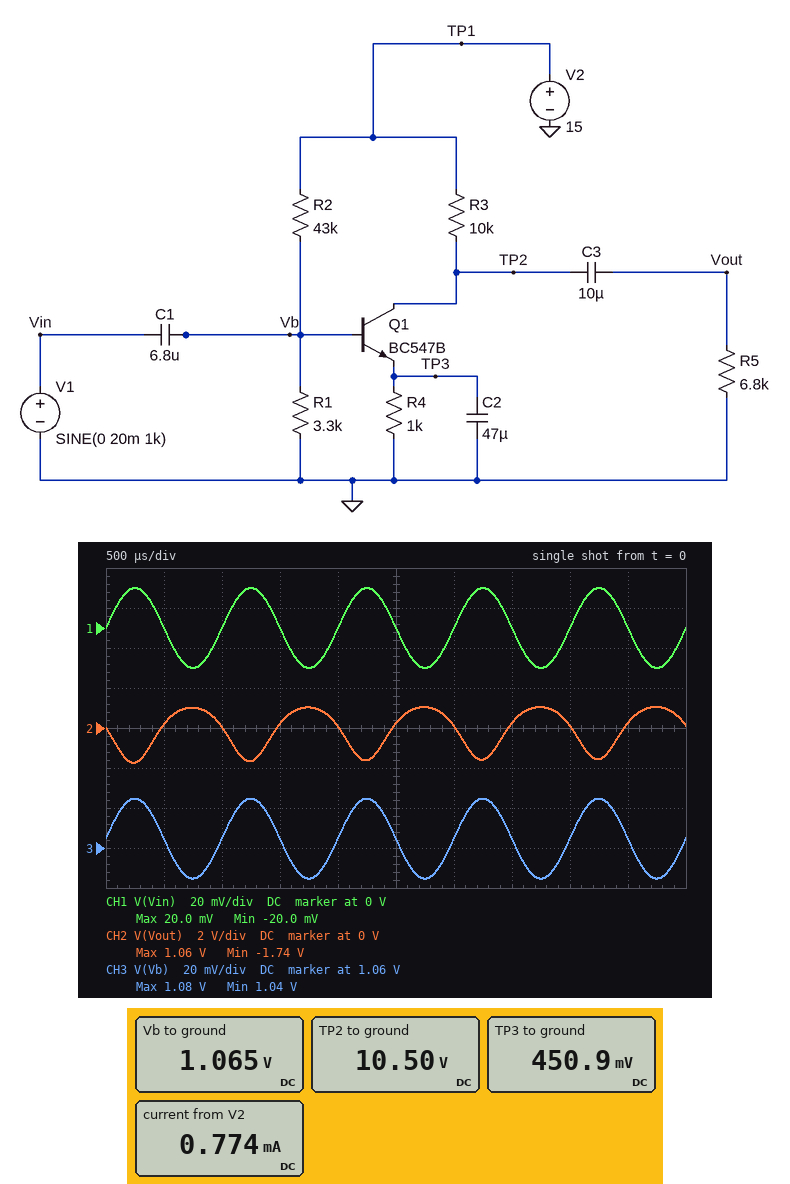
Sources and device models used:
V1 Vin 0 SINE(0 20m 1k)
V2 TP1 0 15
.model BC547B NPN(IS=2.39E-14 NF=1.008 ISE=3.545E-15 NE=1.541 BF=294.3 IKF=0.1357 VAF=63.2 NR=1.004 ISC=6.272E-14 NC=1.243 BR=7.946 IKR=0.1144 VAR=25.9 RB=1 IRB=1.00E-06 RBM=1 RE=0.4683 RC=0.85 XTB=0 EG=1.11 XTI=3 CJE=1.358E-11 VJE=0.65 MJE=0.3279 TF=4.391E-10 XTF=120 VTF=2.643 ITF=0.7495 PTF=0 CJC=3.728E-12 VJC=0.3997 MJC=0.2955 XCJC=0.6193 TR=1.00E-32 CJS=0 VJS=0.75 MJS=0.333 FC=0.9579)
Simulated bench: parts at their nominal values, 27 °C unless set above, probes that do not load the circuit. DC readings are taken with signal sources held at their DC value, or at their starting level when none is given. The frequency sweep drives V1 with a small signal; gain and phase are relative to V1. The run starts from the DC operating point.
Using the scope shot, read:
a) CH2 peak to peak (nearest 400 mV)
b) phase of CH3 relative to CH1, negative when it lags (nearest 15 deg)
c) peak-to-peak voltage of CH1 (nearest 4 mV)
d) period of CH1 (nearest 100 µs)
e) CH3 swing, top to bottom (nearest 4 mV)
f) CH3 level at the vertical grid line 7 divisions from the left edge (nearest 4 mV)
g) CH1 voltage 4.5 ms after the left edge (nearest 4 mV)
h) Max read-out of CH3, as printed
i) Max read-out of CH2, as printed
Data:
2.8 V
0 deg
40 mV
1.0 ms
40 mV
1.064 V
0 V
1.08 V
1.06 V
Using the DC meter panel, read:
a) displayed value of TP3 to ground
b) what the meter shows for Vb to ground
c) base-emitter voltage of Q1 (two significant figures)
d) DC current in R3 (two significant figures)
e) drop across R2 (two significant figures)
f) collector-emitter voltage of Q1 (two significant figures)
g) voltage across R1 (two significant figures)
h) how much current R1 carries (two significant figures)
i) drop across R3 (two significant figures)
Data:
450.9 mV
1.065 V
610 mV
450 µA
14 V
10 V
1.1 V
320 µA
4.5 V
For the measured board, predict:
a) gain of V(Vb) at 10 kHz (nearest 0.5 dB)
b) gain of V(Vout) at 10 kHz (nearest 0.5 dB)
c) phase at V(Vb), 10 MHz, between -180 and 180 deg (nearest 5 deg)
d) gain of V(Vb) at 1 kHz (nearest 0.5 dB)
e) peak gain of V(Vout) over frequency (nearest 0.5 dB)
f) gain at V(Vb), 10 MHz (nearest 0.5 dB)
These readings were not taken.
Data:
0 dB
36.5 dB
0 deg
0 dB
36.5 dB
0 dB
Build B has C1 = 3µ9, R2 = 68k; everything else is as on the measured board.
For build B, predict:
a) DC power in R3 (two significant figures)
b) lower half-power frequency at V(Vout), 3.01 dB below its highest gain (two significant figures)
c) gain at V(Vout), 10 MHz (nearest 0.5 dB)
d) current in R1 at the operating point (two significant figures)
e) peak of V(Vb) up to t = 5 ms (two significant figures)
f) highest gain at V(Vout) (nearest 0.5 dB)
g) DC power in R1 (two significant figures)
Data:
130 µW
25 Hz
24.5 dB
210 µA
710 mV
25.0 dB
150 µW
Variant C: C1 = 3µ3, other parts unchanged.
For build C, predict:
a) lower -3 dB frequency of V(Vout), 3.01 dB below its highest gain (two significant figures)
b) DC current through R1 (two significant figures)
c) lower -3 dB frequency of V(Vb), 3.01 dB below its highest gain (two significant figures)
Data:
66 Hz
320 µA
17 Hz
